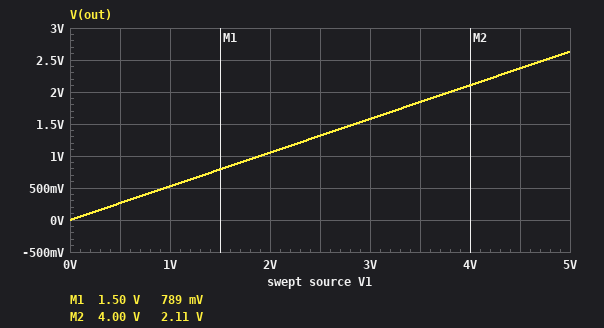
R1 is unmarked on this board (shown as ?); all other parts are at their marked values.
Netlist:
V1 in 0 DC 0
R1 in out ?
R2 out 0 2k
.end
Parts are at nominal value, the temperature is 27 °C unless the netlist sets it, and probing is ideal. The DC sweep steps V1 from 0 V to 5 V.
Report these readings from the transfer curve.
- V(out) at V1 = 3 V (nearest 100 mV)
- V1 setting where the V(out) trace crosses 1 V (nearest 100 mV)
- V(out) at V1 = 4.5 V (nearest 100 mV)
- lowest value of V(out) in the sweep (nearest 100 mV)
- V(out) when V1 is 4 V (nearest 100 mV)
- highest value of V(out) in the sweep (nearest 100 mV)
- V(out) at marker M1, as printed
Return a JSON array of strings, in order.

["1.6 V", "1.9 V", "2.4 V", "0 V", "2.1 V", "2.6 V", "789 mV"]
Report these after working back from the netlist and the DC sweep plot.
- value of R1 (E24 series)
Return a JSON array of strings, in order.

["1.8 kΩ"]
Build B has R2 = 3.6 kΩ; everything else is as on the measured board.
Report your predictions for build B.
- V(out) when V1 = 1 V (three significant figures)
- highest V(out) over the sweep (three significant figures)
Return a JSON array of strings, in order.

["667 mV", "3.33 V"]
